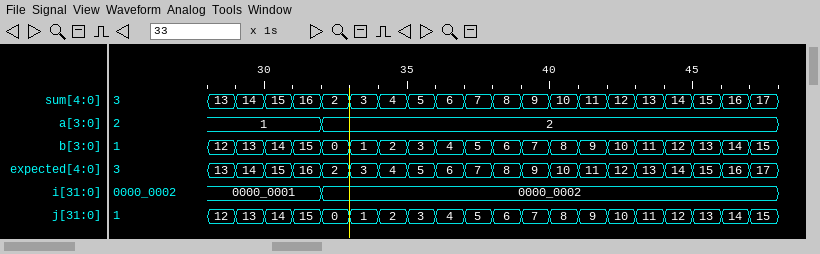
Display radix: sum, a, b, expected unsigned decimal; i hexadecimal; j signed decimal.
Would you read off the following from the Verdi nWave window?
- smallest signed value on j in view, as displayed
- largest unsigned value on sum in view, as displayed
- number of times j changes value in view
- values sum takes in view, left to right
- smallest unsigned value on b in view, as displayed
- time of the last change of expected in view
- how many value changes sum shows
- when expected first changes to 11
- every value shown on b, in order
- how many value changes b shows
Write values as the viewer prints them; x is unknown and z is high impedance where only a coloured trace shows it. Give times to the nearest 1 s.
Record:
0
17
19
13, 14, 15, 16, 2, 3, 4, 5, 6, 7, 8, 9, 10, 11, 12, 13, 14, 15, 16, 17
0
47 s
19
41 s
12, 13, 14, 15, 0, 1, 2, 3, 4, 5, 6, 7, 8, 9, 10, 11, 12, 13, 14, 15
19
